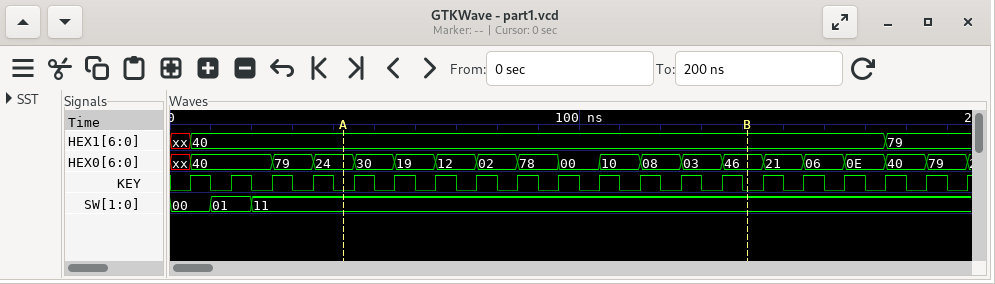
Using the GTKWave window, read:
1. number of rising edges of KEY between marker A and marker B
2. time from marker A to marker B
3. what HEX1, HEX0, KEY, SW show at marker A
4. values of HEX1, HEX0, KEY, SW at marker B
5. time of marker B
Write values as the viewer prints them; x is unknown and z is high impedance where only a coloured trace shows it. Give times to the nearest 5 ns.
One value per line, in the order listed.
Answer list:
10
100 ns
HEX1=40, HEX0=24, KEY=0, SW=11
HEX1=40, HEX0=46, KEY=0, SW=11
140 ns
